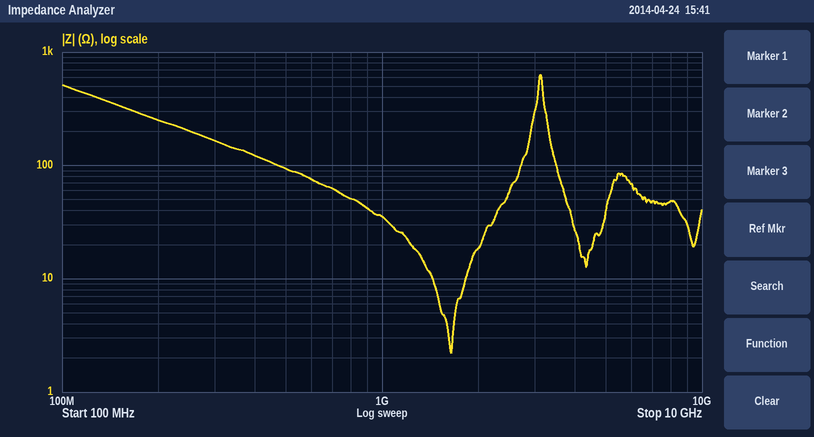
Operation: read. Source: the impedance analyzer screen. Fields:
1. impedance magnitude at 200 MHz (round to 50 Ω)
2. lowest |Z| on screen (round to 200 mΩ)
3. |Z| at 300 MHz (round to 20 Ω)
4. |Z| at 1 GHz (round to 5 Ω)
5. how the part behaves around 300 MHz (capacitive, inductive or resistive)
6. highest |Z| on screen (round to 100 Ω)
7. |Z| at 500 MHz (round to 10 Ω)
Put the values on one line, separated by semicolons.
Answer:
250 Ω; 2.2 Ω; 160 Ω; 35 Ω; capacitive; 600 Ω; 90 Ω
